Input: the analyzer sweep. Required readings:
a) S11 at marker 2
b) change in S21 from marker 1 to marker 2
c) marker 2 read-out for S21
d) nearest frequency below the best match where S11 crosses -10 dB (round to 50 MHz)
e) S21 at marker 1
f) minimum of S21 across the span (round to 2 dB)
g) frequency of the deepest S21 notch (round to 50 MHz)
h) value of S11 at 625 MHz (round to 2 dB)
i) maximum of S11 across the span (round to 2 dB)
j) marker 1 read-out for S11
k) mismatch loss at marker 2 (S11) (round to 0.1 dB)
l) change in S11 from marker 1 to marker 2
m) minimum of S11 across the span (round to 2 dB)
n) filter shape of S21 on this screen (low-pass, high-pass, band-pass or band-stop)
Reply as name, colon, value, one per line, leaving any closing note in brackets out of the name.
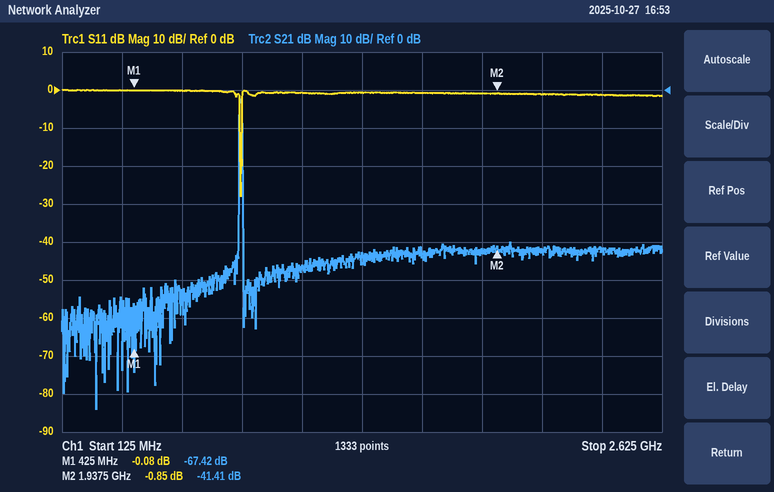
S11 at marker 2: -0.85 dB
change in S21 from marker 1 to marker 2: 26.01 dB
marker 2 read-out for S21: -41.41 dB
nearest frequency below the best match where S11 crosses -10 dB: 850 MHz
S21 at marker 1: -67.42 dB
minimum of S21 across the span: -84 dB
frequency of the deepest S21 notch: 250 MHz
value of S11 at 625 MHz: 0 dB
maximum of S11 across the span: 0 dB
marker 1 read-out for S11: -0.08 dB
mismatch loss at marker 2 (S11): 7.5 dB
change in S11 from marker 1 to marker 2: -0.77 dB
minimum of S11 across the span: -28 dB
filter shape of S21 on this screen: band-pass
